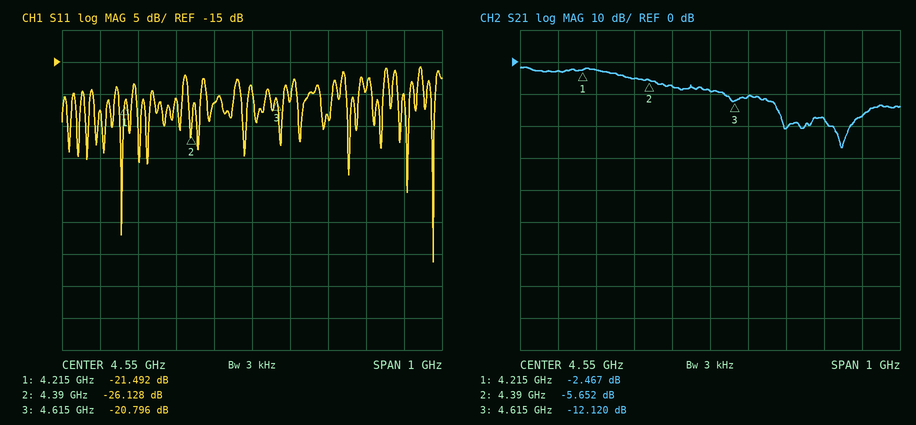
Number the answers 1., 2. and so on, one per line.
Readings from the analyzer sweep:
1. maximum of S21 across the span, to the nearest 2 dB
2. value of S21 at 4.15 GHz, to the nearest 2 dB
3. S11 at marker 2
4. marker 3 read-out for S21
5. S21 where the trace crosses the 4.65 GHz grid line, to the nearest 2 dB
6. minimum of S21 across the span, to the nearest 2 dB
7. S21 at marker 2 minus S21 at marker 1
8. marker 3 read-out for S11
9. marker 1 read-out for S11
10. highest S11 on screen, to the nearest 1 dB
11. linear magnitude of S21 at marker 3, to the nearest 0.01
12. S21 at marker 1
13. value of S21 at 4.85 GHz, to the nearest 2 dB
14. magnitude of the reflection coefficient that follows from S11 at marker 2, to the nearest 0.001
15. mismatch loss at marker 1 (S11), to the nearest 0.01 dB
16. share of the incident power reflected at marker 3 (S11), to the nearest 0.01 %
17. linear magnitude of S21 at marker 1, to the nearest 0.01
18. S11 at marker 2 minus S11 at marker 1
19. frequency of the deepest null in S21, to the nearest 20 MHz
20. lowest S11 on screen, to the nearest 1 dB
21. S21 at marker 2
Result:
1. -2 dB
2. -2 dB
3. -26.128 dB
4. -12.120 dB
5. -10 dB
6. -26 dB
7. -3.185 dB
8. -20.796 dB
9. -21.492 dB
10. -16 dB
11. 0.25
12. -2.467 dB
13. -18 dB
14. 0.049
15. 0.03 dB
16. 0.83 %
17. 0.75
18. -4.636 dB
19. 4.90 GHz
20. -46 dB
21. -5.652 dB
